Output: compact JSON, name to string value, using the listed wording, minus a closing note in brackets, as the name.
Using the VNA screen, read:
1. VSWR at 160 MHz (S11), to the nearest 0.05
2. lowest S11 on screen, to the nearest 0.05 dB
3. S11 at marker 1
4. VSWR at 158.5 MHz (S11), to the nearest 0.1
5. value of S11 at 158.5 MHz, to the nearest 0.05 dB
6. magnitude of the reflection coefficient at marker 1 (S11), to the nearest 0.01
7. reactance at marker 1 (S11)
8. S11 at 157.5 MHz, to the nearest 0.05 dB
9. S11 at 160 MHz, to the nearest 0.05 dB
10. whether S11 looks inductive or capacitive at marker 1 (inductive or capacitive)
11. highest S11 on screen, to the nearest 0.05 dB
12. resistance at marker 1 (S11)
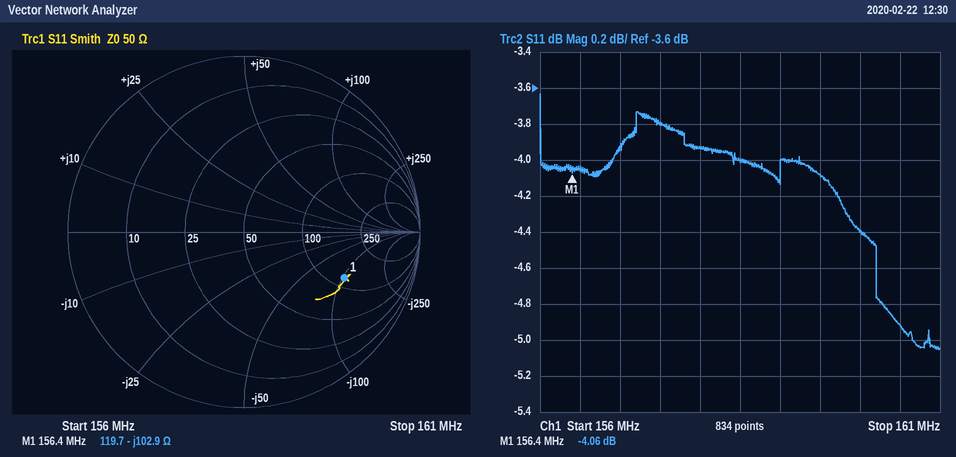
{"VSWR at 160 MHz (S11), to the nearest 0.05": "4.05", "lowest S11 on screen, to the nearest 0.05 dB": "-5.05 dB", "S11 at marker 1": "-4.06 dB", "VSWR at 158.5 MHz (S11), to the nearest 0.1": "4.4", "value of S11 at 158.5 MHz, to the nearest 0.05 dB": "-4.00 dB", "magnitude of the reflection coefficient at marker 1 (S11), to the nearest 0.01": "0.63", "reactance at marker 1": "-102.9 Ω", "S11 at 157.5 MHz, to the nearest 0.05 dB": "-3.80 dB", "S11 at 160 MHz, to the nearest 0.05 dB": "-4.40 dB", "whether S11 looks inductive or capacitive at marker 1": "capacitive", "highest S11 on screen, to the nearest 0.05 dB": "-3.65 dB", "resistance at marker 1": "119.7 Ω"}
